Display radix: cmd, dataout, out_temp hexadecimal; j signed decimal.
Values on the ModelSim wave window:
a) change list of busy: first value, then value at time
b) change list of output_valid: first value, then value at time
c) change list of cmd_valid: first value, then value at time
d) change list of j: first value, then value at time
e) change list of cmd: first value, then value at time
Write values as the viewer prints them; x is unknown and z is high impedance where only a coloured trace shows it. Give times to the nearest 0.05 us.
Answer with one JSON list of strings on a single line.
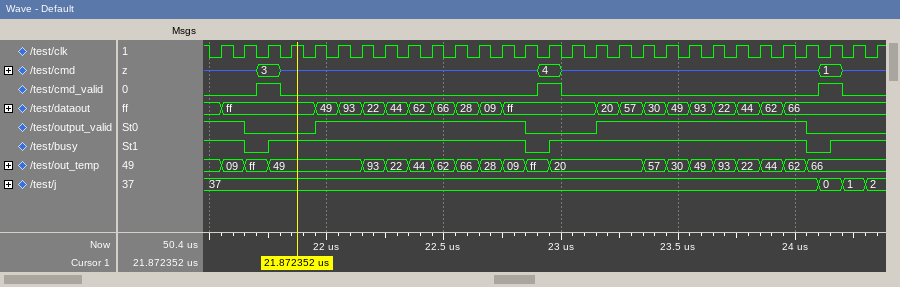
["1, 0 at 21.65 us, 1 at 21.75 us, 0 at 22.85 us, 1 at 22.95 us, 0 at 24.05 us, 1 at 24.15 us", "1, 0 at 21.65 us, 1 at 21.95 us, 0 at 22.85 us, 1 at 23.15 us, 0 at 24.05 us", "0, 1 at 21.7 us, 0 at 21.8 us, 1 at 22.9 us, 0 at 23 us, 1 at 24.1 us, 0 at 24.2 us", "37, 0 at 24.1 us, 1 at 24.2 us, 2 at 24.3 us", "z, 3 at 21.7 us, z at 21.8 us, 4 at 22.9 us, z at 23 us, 1 at 24.1 us, z at 24.2 us"]
